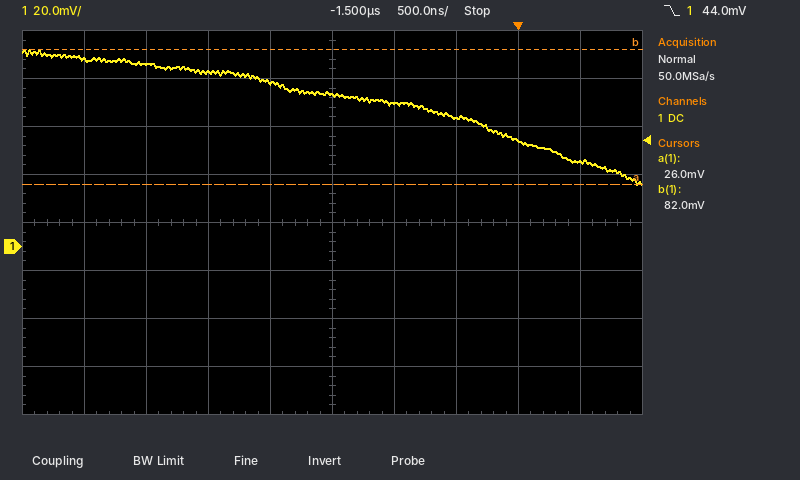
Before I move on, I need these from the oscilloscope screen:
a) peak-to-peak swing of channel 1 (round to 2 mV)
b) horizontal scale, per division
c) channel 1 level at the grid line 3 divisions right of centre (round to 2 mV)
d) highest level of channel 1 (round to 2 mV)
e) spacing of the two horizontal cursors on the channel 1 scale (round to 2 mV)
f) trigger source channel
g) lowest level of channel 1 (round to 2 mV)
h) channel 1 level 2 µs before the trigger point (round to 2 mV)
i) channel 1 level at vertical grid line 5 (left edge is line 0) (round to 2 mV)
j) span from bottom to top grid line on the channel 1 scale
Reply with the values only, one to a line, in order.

56 mV
500 ns
44 mV
82 mV
56 mV
channel 1
26 mV
68 mV
64 mV
160 mV
